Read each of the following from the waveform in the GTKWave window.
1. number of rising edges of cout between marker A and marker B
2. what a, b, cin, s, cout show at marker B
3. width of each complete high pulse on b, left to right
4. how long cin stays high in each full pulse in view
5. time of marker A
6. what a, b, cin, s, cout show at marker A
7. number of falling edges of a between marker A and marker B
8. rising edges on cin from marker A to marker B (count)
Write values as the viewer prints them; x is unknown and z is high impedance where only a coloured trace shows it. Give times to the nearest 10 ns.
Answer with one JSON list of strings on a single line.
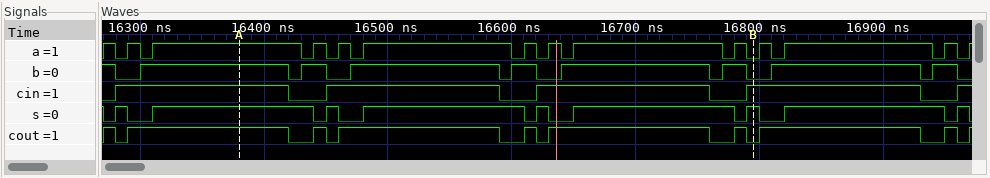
["5", "a=0, b=0, cin=1, s=1, cout=0", "120 ns, 20 ns, 120 ns, 20 ns, 120 ns, 20 ns, 120 ns, 20 ns", "140 ns, 140 ns, 140 ns, 140 ns", "16380 ns", "a=1, b=1, cin=1, s=1, cout=1", "8", "3"]
